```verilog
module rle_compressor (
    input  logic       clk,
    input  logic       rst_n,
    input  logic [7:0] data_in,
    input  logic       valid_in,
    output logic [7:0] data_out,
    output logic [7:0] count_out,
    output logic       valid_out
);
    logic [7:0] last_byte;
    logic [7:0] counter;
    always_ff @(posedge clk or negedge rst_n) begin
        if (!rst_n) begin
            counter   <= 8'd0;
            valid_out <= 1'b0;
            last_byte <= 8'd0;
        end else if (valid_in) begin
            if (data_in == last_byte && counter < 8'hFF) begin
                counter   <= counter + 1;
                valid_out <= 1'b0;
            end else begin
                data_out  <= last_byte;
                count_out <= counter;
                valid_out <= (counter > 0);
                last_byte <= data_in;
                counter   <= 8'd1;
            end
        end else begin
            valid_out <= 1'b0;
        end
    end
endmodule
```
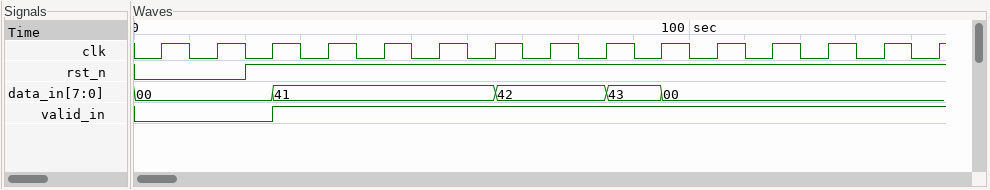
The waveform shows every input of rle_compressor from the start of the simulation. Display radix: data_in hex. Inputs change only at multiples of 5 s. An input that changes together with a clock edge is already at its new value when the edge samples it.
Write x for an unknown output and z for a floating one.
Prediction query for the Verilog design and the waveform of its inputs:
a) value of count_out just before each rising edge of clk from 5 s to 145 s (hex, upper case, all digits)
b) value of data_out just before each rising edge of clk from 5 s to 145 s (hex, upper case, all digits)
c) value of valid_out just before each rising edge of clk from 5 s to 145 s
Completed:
x, x, x, 00, 00, 00, 00, 04, 04, 02, 01, 01, 01, 01, 01
x, x, x, 00, 00, 00, 00, 41, 41, 42, 43, 43, 43, 43, 43
0 0 0 0 0 0 0 1 0 1 1 0 0 0 0
